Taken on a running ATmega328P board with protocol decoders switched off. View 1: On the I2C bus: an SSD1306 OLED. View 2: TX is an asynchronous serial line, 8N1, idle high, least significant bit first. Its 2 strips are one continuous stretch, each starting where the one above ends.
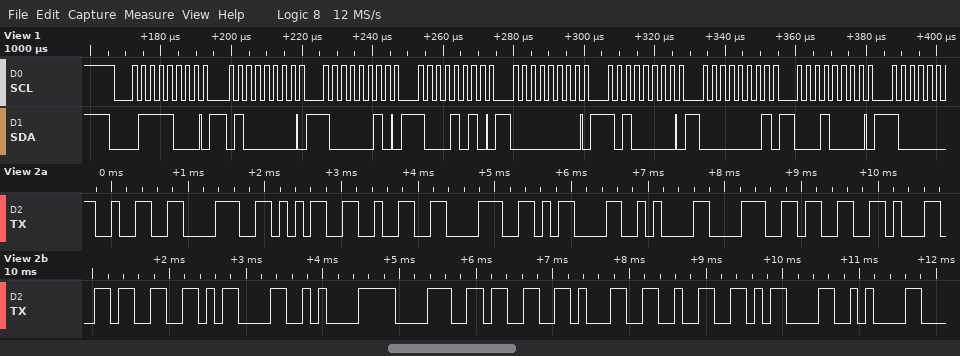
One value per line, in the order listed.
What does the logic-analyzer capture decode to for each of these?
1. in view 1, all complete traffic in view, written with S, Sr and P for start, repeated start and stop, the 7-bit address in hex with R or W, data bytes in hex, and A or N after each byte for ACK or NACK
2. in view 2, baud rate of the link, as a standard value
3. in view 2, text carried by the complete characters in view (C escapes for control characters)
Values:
S 3CW A 40 A 82 A 8A A 00 A A0 A 01 A 10 A
9600 baud
"28528\r\n8313\r\n8312\r\n"
